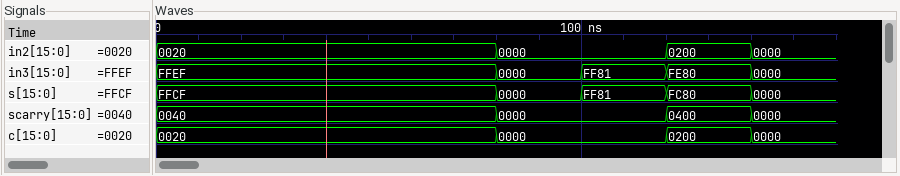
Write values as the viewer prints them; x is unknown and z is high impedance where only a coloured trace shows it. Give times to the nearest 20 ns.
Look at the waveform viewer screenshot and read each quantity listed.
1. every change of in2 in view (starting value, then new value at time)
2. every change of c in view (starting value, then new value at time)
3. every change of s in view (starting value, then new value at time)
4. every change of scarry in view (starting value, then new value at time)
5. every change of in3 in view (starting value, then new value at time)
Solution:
0020, 0000 at 80 ns, 0200 at 120 ns, 0000 at 140 ns
0020, 0000 at 80 ns, 0200 at 120 ns, 0000 at 140 ns
FFCF, 0000 at 80 ns, FF81 at 100 ns, FC80 at 120 ns, 0000 at 140 ns
0040, 0000 at 80 ns, 0400 at 120 ns, 0000 at 140 ns
FFEF, 0000 at 80 ns, FF81 at 100 ns, FE80 at 120 ns, 0000 at 140 ns
